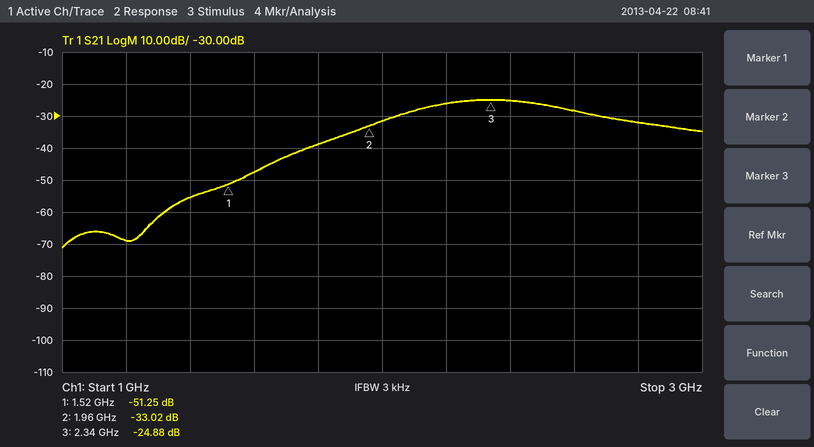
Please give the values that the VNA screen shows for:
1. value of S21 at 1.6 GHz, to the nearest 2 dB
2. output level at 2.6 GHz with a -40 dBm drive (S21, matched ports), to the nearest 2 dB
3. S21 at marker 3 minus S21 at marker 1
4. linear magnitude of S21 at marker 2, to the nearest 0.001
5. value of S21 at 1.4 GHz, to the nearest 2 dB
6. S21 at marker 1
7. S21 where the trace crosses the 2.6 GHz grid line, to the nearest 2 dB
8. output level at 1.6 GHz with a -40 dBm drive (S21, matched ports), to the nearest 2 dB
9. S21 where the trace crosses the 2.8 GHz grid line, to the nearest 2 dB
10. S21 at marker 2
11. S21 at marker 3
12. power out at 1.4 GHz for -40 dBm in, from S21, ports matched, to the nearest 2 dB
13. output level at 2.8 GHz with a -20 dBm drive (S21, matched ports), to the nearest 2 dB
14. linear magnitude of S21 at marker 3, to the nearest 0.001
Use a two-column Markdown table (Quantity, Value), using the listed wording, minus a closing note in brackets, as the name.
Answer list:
| Quantity | Value |
|---|---|
| value of S21 at 1.6 GHz, to the nearest 2 dB | -48 dB |
| output level at 2.6 GHz with a -40 dBm drive (S21, matched ports), to the nearest 2 dB | -68 dBm |
| S21 at marker 3 minus S21 at marker 1 | 26.37 dB |
| linear magnitude of S21 at marker 2, to the nearest 0.001 | 0.022 |
| value of S21 at 1.4 GHz, to the nearest 2 dB | -56 dB |
| S21 at marker 1 | -51.25 dB |
| S21 where the trace crosses the 2.6 GHz grid line, to the nearest 2 dB | -28 dB |
| output level at 1.6 GHz with a -40 dBm drive (S21, matched ports), to the nearest 2 dB | -88 dBm |
| S21 where the trace crosses the 2.8 GHz grid line, to the nearest 2 dB | -32 dB |
| S21 at marker 2 | -33.02 dB |
| S21 at marker 3 | -24.88 dB |
| power out at 1.4 GHz for -40 dBm in, from S21, ports matched, to the nearest 2 dB | -96 dBm |
| output level at 2.8 GHz with a -20 dBm drive (S21, matched ports), to the nearest 2 dB | -52 dBm |
| linear magnitude of S21 at marker 3, to the nearest 0.001 | 0.057 |
